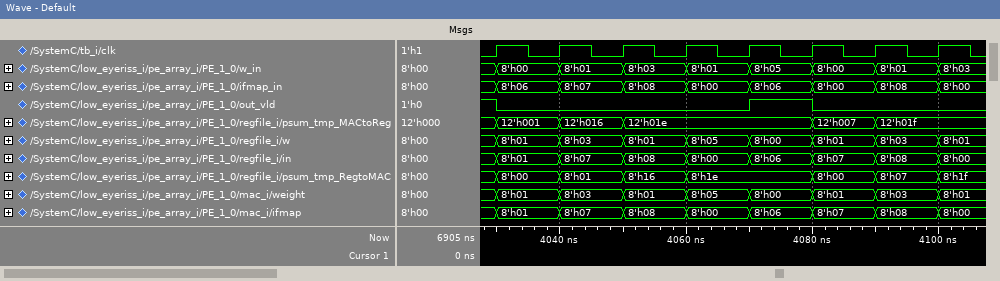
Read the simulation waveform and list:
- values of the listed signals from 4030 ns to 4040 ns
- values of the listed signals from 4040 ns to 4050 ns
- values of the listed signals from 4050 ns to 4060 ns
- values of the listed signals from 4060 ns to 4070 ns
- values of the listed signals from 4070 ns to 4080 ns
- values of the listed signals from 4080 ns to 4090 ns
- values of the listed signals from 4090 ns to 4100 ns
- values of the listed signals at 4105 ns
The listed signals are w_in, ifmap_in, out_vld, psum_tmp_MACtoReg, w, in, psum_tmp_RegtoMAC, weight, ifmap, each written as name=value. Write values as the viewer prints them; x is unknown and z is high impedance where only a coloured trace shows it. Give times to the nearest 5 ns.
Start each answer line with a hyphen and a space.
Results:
- w_in=8'h00, ifmap_in=8'h06, out_vld=0, psum_tmp_MACtoReg=12'h001, w=8'h01, in=8'h01, psum_tmp_RegtoMAC=8'h00, weight=8'h01, ifmap=8'h01
- w_in=8'h01, ifmap_in=8'h07, out_vld=0, psum_tmp_MACtoReg=12'h016, w=8'h03, in=8'h07, psum_tmp_RegtoMAC=8'h01, weight=8'h03, ifmap=8'h07
- w_in=8'h03, ifmap_in=8'h08, out_vld=0, psum_tmp_MACtoReg=12'h01e, w=8'h01, in=8'h08, psum_tmp_RegtoMAC=8'h16, weight=8'h01, ifmap=8'h08
- w_in=8'h01, ifmap_in=8'h00, out_vld=0, psum_tmp_MACtoReg=12'h01e, w=8'h05, in=8'h00, psum_tmp_RegtoMAC=8'h1e, weight=8'h05, ifmap=8'h00
- w_in=8'h05, ifmap_in=8'h06, out_vld=1, psum_tmp_MACtoReg=12'h01e, w=8'h00, in=8'h06, psum_tmp_RegtoMAC=8'h1e, weight=8'h00, ifmap=8'h06
- w_in=8'h00, ifmap_in=8'h00, out_vld=0, psum_tmp_MACtoReg=12'h007, w=8'h01, in=8'h07, psum_tmp_RegtoMAC=8'h00, weight=8'h01, ifmap=8'h07
- w_in=8'h01, ifmap_in=8'h08, out_vld=0, psum_tmp_MACtoReg=12'h01f, w=8'h03, in=8'h08, psum_tmp_RegtoMAC=8'h07, weight=8'h03, ifmap=8'h08
- w_in=8'h03, ifmap_in=8'h00, out_vld=0, psum_tmp_MACtoReg=12'h01f, w=8'h01, in=8'h00, psum_tmp_RegtoMAC=8'h1f, weight=8'h01, ifmap=8'h00
